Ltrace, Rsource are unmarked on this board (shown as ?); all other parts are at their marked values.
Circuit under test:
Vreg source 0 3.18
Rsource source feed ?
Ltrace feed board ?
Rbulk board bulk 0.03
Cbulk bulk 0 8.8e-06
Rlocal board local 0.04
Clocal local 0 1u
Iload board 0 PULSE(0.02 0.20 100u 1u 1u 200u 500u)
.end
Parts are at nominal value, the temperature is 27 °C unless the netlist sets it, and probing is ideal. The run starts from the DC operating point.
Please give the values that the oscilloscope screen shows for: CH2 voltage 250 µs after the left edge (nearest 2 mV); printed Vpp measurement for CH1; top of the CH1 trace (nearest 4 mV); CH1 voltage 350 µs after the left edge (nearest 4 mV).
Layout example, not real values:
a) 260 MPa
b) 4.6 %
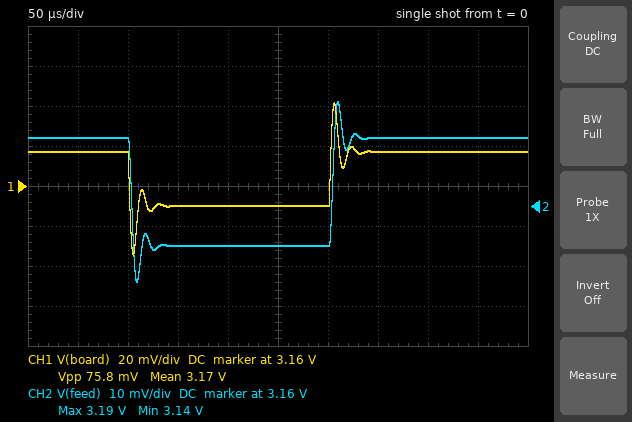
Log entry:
a) 3.150 V
b) 75.8 mV
c) 3.200 V
d) 3.176 V
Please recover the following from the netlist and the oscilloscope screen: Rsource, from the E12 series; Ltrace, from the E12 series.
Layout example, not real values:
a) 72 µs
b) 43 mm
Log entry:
a) 0.15 Ω
b) 680 nH
